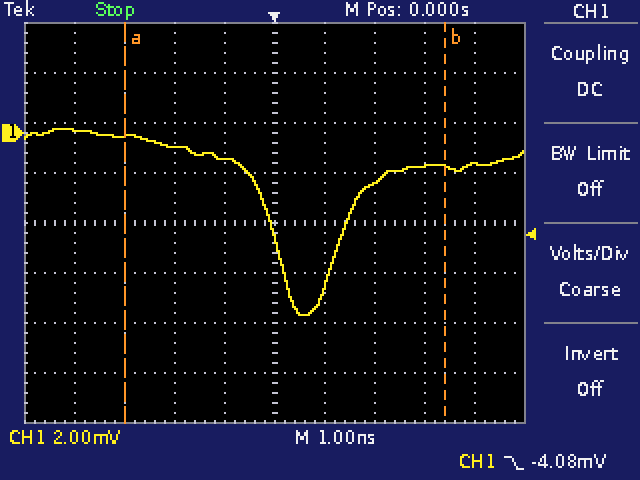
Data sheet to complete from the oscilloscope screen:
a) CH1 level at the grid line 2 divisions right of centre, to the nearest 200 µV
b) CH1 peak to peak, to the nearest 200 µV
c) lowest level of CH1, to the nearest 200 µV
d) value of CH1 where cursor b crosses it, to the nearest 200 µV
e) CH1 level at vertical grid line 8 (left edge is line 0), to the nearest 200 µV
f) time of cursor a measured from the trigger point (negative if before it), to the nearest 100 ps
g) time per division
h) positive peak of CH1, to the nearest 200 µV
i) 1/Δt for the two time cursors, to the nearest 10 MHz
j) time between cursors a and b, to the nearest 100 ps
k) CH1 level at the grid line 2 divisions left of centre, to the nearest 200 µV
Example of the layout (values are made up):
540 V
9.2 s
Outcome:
-2.0 mV
7.4 mV
-7.2 mV
-1.4 mV
-1.4 mV
-3.0 ns
1 ns
200 µV
160 MHz
6.4 ns
-600 µV
